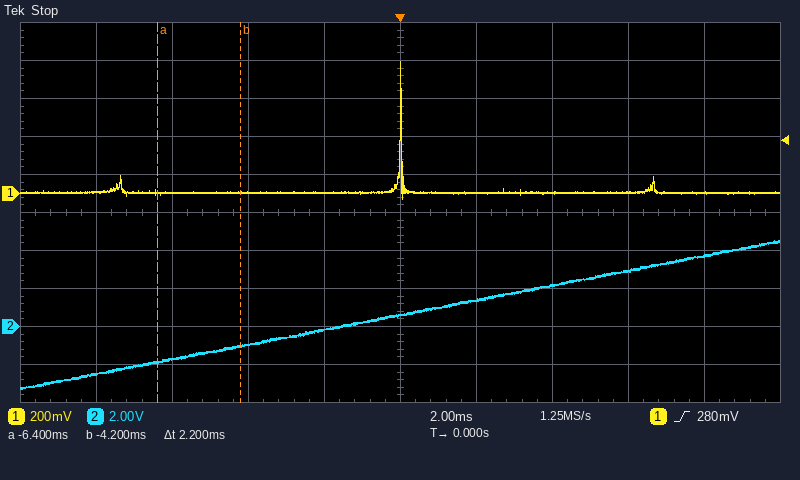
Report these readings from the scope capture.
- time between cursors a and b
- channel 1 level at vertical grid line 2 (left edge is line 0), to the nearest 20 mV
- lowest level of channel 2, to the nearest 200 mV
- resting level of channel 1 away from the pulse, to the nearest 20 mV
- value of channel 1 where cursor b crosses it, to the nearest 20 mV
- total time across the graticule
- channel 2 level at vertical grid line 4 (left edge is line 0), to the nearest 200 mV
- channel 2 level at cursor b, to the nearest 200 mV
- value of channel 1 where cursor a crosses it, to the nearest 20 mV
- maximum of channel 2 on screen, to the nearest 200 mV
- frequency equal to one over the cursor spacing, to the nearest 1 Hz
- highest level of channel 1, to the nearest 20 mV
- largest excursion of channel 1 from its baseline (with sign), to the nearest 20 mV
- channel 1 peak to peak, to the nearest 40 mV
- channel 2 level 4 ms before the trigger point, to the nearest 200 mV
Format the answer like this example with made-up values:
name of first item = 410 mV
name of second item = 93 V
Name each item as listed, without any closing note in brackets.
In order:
time between cursors a and b = 2.2 ms
channel 1 level at vertical grid line 2 (left edge is line 0), to the nearest 20 mV = 0 mV
lowest level of channel 2, to the nearest 200 mV = -3.4 V
resting level of channel 1 away from the pulse, to the nearest 20 mV = 0 mV
value of channel 1 where cursor b crosses it, to the nearest 20 mV = 0 mV
total time across the graticule = 20 ms
channel 2 level at vertical grid line 4 (left edge is line 0), to the nearest 200 mV = -200 mV
channel 2 level at cursor b, to the nearest 200 mV = -1.0 V
value of channel 1 where cursor a crosses it, to the nearest 20 mV = 0 mV
maximum of channel 2 on screen, to the nearest 200 mV = 4.6 V
frequency equal to one over the cursor spacing, to the nearest 1 Hz = 455 Hz
highest level of channel 1, to the nearest 20 mV = 700 mV
largest excursion of channel 1 from its baseline (with sign), to the nearest 20 mV = +700 mV
channel 1 peak to peak, to the nearest 40 mV = 720 mV
channel 2 level 4 ms before the trigger point, to the nearest 200 mV = -1.0 V
